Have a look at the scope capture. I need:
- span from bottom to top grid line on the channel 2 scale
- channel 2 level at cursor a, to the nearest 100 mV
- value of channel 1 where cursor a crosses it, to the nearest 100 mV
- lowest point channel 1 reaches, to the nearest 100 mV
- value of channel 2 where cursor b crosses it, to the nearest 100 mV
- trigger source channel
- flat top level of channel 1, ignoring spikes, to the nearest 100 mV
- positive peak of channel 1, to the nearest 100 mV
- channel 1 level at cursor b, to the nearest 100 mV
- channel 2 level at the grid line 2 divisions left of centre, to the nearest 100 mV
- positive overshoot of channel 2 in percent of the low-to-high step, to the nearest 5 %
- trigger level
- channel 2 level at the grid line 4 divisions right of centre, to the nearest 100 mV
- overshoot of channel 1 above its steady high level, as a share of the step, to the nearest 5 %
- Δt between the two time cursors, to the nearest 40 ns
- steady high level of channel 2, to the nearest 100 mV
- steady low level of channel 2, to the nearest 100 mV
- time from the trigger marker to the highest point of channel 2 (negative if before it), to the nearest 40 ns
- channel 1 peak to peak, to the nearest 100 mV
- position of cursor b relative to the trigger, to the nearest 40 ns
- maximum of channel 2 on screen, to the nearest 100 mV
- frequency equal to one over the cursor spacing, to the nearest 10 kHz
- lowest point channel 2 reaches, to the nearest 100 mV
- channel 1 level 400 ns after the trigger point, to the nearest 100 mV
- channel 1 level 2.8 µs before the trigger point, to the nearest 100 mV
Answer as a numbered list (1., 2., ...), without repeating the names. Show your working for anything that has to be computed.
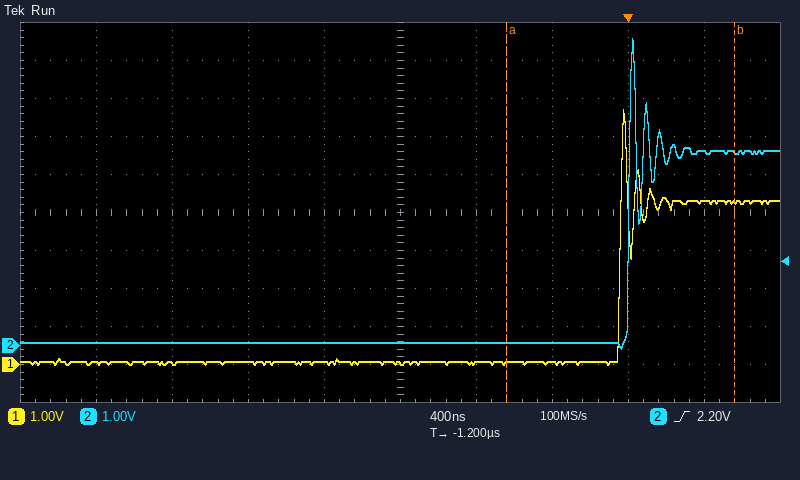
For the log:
1. 10 V
2. 100 mV
3. 0.0 V
4. 0.0 V
5. 5.1 V
6. channel 2
7. 4.3 V
8. 6.7 V
9. 4.3 V
10. 100 mV
11. 60 %
12. 2.20 V
13. 5.1 V
14. 55 %
15. 1.20 µs
16. 5.1 V
17. 100 mV
18. +40 ns
19. 6.7 V − (0.0 V) = 6.7 V
20. +560 ns
21. 8.1 V
22. 1 / 1.20 µs ≈ 830 kHz
23. -100 mV
24. 4.3 V
25. 0.0 V
